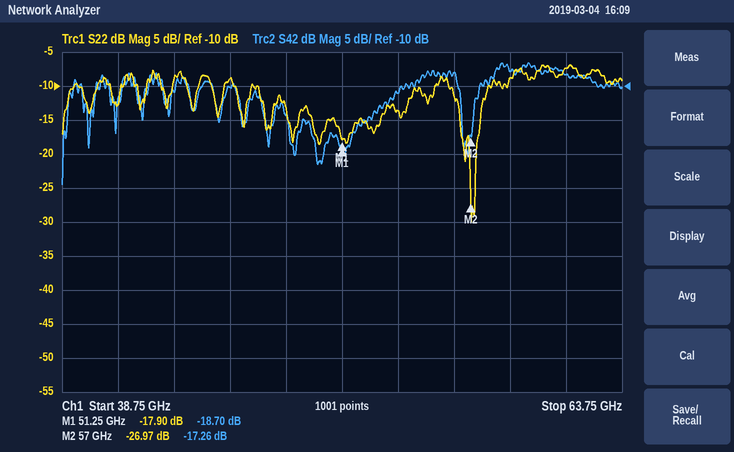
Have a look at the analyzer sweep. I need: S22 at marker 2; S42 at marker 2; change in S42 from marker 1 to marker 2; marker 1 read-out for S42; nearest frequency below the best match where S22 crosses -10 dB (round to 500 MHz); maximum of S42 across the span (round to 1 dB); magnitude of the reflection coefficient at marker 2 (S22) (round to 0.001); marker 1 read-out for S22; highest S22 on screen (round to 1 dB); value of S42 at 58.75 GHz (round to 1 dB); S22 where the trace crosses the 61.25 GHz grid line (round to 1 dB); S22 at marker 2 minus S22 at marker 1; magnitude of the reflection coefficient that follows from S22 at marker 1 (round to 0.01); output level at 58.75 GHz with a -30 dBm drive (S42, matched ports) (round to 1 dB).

-26.97 dB
-17.26 dB
1.44 dB
-18.70 dB
56.0 GHz
-7 dB
0.045
-17.90 dB
-7 dB
-8 dB
-7 dB
-9.07 dB
0.13
-38 dBm
